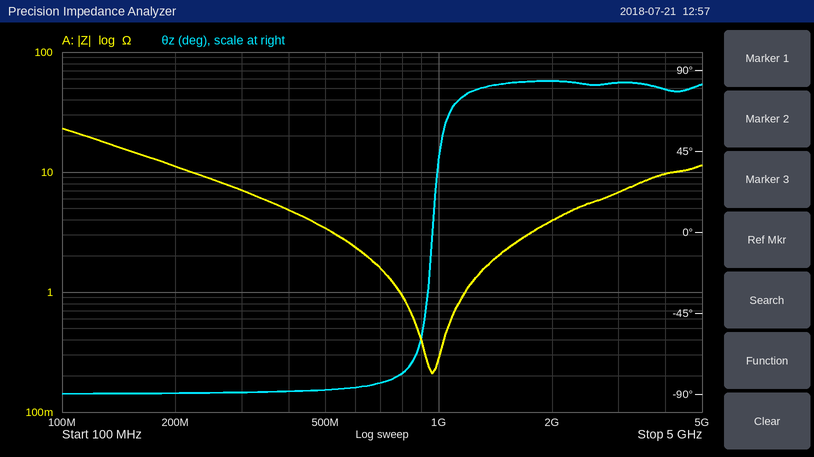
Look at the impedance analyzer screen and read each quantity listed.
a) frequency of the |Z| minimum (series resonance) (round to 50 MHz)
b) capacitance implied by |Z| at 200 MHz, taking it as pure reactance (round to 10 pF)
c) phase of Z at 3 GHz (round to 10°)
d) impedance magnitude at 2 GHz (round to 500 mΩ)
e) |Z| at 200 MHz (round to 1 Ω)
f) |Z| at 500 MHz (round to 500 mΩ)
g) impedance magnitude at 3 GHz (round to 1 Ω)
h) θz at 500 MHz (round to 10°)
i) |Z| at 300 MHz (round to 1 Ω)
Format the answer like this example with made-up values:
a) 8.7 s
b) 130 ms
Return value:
a) 950 MHz
b) 70 pF
c) 80°
d) 4.0 Ω
e) 11 Ω
f) 3.5 Ω
g) 7 Ω
h) -90°
i) 7 Ω
